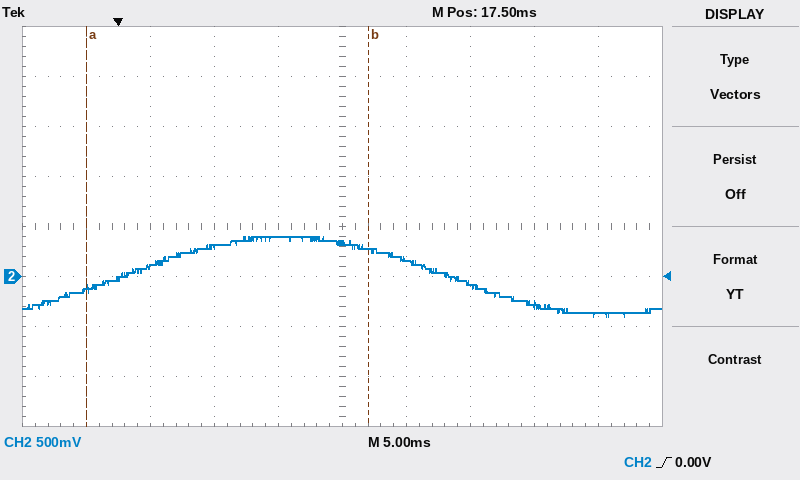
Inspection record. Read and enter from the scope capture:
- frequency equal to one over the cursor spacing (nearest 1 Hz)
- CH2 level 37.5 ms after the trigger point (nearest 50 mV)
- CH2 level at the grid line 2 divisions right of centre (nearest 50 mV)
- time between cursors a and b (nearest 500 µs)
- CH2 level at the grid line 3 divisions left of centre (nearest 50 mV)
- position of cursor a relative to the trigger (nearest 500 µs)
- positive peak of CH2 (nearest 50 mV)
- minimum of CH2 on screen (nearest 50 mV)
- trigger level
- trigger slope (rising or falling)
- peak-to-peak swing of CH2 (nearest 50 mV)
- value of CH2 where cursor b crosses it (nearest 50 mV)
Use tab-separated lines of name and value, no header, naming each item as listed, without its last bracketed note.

frequency equal to one over the cursor spacing	45 Hz
CH2 level 37.5 ms after the trigger point	-350 mV
CH2 level at the grid line 2 divisions right of centre	-100 mV
time between cursors a and b	22.0 ms
CH2 level at the grid line 3 divisions left of centre	100 mV
position of cursor a relative to the trigger	-2.5 ms
positive peak of CH2	400 mV
minimum of CH2 on screen	-400 mV
trigger level	0.00 V
trigger slope	rising
peak-to-peak swing of CH2	800 mV
value of CH2 where cursor b crosses it	250 mV
